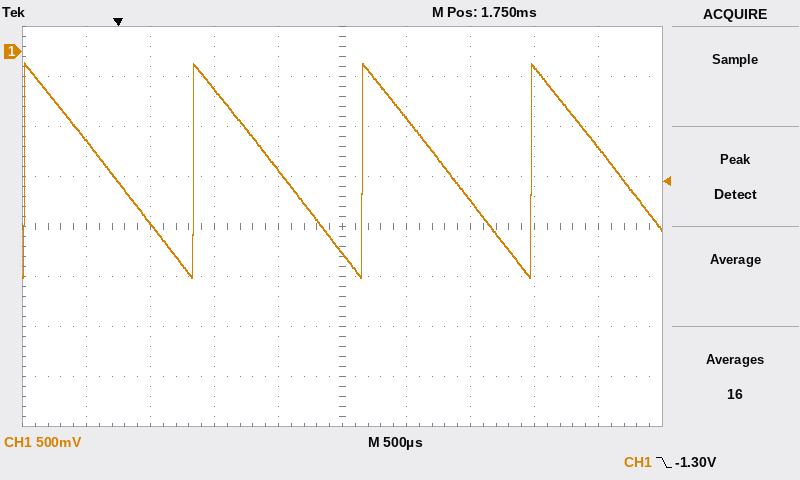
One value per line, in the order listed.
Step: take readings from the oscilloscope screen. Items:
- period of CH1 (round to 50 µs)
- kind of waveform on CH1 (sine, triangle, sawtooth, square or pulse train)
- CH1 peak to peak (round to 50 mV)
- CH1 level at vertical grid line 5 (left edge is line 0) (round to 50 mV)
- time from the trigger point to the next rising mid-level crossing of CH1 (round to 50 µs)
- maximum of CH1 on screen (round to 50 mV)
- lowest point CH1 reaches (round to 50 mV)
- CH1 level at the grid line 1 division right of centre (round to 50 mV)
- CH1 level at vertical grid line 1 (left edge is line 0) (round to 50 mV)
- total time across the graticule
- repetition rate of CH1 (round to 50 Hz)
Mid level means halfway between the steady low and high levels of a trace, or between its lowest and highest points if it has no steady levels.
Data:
1.30 ms
sawtooth
2.15 V
-2.00 V
600 µs
-100 mV
-2.25 V
-650 mV
-900 mV
5 ms
750 Hz
